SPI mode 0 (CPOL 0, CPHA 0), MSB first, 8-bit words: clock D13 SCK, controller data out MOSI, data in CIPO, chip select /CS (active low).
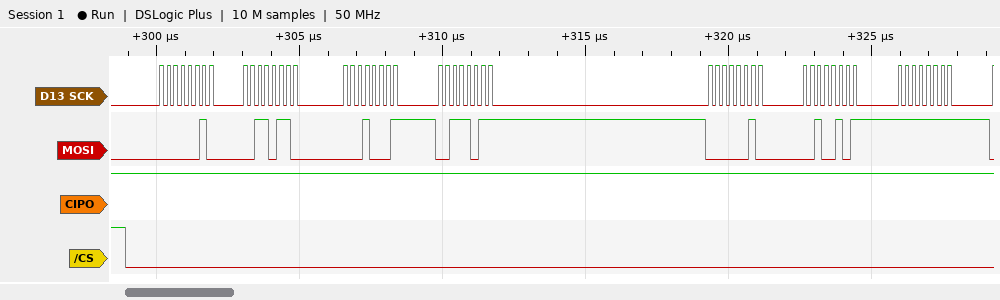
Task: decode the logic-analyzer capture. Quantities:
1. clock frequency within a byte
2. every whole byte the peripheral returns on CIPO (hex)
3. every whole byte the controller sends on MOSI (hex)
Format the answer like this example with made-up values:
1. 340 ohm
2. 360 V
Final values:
1. 4 MHz
2. FF FF FF FF FF FF FF
3. 02 36 11 3B 02 25 FF
